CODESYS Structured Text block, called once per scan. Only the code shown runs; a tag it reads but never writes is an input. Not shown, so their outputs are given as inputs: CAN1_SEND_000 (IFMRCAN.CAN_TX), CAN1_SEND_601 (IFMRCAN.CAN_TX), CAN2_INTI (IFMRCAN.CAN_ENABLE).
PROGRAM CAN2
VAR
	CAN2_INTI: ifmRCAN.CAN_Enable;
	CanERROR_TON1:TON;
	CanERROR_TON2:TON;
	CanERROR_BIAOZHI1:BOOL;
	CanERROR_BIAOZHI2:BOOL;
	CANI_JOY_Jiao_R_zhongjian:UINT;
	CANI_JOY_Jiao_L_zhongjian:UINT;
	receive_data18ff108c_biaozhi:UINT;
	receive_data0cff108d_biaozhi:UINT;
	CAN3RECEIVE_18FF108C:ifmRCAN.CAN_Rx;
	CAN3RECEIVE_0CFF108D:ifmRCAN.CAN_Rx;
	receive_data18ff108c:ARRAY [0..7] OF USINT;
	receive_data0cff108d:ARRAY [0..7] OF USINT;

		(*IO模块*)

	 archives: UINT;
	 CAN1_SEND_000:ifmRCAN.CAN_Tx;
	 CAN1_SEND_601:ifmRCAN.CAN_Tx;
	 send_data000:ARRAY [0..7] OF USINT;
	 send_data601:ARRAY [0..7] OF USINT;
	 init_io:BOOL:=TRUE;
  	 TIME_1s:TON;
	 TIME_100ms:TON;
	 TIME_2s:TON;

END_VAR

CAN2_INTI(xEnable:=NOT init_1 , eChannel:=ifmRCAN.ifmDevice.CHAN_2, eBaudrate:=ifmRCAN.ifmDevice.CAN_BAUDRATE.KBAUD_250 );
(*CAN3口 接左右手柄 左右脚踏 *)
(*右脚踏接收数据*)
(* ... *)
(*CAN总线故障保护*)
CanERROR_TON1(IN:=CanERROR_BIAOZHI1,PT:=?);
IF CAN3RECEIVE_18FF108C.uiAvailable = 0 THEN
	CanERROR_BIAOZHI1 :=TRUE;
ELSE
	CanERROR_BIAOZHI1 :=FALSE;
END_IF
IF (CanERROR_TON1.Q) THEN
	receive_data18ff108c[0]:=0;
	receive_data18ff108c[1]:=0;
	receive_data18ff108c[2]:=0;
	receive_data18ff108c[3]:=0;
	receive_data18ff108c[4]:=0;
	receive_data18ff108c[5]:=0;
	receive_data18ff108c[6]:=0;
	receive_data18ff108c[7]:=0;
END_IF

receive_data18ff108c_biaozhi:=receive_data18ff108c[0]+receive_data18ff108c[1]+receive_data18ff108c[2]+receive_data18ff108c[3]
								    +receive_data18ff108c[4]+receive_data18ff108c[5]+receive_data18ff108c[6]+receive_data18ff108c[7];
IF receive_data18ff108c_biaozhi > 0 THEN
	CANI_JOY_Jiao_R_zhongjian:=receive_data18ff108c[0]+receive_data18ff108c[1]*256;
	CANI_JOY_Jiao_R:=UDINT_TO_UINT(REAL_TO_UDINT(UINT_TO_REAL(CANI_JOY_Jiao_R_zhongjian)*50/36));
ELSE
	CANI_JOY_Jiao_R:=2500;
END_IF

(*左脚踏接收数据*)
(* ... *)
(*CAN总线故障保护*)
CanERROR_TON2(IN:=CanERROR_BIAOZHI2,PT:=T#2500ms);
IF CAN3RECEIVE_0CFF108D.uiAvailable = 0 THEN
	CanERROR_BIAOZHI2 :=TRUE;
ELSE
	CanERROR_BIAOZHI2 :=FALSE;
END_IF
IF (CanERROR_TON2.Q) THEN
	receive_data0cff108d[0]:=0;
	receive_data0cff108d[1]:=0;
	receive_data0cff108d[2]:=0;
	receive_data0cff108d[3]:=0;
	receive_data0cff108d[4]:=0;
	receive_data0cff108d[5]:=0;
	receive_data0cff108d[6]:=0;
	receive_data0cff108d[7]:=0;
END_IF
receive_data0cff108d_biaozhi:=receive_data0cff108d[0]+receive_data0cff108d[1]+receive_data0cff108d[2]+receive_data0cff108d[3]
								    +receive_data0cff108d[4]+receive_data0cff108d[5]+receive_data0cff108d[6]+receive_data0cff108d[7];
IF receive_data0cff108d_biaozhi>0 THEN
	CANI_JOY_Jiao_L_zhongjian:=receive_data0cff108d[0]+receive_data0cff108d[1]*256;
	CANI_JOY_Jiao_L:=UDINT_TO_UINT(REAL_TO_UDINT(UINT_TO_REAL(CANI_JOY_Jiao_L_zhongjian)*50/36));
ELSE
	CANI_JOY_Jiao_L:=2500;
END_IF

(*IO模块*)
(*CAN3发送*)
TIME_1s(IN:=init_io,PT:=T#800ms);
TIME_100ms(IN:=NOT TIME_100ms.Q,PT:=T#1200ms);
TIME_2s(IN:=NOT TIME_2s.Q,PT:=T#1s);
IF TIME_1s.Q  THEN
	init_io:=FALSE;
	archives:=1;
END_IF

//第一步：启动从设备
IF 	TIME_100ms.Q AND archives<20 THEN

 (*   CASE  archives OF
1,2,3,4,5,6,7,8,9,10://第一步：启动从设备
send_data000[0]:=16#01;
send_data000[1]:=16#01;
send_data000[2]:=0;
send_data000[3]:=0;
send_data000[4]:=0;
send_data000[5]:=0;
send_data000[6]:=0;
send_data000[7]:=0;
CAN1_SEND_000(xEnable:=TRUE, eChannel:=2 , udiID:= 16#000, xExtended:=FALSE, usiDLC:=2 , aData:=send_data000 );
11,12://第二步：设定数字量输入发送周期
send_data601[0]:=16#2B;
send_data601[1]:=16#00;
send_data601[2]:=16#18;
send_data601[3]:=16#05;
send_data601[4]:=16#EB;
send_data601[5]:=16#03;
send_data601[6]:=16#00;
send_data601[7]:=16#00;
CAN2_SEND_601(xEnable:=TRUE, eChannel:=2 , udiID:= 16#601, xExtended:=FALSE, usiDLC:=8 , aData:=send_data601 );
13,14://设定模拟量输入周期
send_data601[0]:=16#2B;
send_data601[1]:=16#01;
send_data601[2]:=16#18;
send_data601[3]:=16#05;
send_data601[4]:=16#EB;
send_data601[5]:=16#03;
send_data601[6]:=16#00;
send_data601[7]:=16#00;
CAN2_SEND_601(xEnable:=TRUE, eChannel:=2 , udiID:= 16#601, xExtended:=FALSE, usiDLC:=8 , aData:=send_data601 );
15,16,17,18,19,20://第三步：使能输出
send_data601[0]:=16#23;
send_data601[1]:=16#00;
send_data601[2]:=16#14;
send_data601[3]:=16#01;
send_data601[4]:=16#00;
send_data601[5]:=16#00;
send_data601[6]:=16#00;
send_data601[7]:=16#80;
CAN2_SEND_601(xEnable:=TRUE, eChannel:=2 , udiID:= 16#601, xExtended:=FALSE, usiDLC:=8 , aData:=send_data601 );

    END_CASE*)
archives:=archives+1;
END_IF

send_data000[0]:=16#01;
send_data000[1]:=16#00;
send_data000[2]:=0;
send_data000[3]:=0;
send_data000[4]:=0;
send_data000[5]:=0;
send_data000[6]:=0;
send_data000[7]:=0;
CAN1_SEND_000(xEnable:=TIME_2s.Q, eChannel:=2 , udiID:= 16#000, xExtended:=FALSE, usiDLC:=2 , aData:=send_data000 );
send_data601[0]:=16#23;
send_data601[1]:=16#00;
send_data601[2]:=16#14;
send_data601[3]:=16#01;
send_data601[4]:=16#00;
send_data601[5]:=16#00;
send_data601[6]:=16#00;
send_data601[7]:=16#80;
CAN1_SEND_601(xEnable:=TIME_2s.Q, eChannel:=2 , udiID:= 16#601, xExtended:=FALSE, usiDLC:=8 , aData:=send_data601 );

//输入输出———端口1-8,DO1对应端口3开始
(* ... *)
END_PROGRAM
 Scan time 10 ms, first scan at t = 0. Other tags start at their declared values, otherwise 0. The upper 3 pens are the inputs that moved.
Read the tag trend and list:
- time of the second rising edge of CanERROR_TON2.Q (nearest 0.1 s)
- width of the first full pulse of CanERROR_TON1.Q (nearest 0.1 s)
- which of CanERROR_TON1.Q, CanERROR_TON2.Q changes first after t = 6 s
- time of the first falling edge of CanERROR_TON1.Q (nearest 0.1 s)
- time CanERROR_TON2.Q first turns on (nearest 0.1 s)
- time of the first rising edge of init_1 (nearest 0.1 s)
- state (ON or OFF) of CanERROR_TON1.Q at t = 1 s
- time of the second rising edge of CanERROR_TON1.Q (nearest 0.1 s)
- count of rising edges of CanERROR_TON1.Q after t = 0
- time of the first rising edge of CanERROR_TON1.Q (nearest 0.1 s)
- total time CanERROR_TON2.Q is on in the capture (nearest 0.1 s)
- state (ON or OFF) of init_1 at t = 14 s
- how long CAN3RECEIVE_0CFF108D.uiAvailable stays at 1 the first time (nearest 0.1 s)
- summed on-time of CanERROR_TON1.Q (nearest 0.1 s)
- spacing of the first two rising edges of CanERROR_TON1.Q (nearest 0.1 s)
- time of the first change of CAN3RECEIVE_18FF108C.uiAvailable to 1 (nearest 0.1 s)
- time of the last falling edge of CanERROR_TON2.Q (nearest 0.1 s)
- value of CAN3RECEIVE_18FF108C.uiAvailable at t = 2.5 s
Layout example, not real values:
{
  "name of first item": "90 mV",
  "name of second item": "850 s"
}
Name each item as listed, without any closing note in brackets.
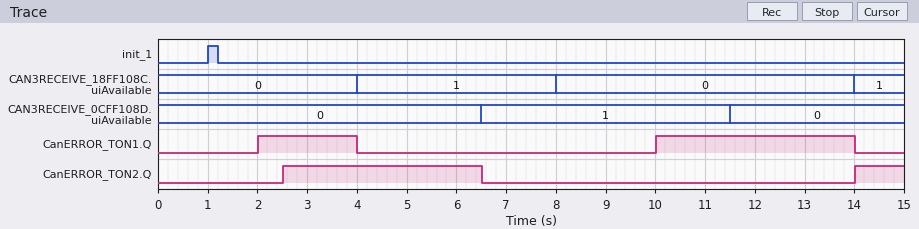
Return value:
{
  "time of the second rising edge of CanERROR_TON2.Q": "14.0 s",
  "width of the first full pulse of CanERROR_TON1.Q": "2.0 s",
  "which of CanERROR_TON1.Q, CanERROR_TON2.Q changes first after t = 6 s": "CanERROR_TON2.Q",
  "time of the first falling edge of CanERROR_TON1.Q": "4.0 s",
  "time CanERROR_TON2.Q first turns on": "2.5 s",
  "time of the first rising edge of init_1": "1.0 s",
  "state (ON or OFF) of CanERROR_TON1.Q at t = 1 s": "OFF",
  "time of the second rising edge of CanERROR_TON1.Q": "10.0 s",
  "count of rising edges of CanERROR_TON1.Q after t = 0": "2",
  "time of the first rising edge of CanERROR_TON1.Q": "2.0 s",
  "total time CanERROR_TON2.Q is on in the capture": "5.0 s",
  "state (ON or OFF) of init_1 at t = 14 s": "OFF",
  "how long CAN3RECEIVE_0CFF108D.uiAvailable stays at 1 the first time": "5.0 s",
  "summed on-time of CanERROR_TON1.Q": "6.0 s",
  "spacing of the first two rising edges of CanERROR_TON1.Q": "8.0 s",
  "time of the first change of CAN3RECEIVE_18FF108C.uiAvailable to 1": "4.0 s",
  "time of the last falling edge of CanERROR_TON2.Q": "6.5 s",
  "value of CAN3RECEIVE_18FF108C.uiAvailable at t = 2.5 s": "0"
}
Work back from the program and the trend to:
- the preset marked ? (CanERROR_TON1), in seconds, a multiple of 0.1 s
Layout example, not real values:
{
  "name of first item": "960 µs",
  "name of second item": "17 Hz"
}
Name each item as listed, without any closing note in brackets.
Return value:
{
  "the preset marked ? (CanERROR_TON1), in seconds, a multiple of 0.1 s": "2.0 s"
}
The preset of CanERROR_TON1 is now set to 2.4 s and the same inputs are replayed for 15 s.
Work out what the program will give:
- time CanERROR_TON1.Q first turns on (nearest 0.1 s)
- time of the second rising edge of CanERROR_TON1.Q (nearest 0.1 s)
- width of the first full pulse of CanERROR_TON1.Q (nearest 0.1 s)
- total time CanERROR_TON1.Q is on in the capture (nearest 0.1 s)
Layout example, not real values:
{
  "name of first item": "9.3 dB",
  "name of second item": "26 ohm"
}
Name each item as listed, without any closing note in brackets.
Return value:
{
  "time CanERROR_TON1.Q first turns on": "2.4 s",
  "time of the second rising edge of CanERROR_TON1.Q": "10.4 s",
  "width of the first full pulse of CanERROR_TON1.Q": "1.6 s",
  "total time CanERROR_TON1.Q is on in the capture": "5.2 s"
}
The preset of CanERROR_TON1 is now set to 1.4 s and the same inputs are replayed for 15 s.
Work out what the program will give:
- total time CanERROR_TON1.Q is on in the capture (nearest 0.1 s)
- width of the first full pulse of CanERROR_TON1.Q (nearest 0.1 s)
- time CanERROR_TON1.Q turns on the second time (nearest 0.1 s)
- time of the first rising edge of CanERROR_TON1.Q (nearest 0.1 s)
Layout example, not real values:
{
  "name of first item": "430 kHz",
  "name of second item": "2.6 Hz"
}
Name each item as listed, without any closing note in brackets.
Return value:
{
  "total time CanERROR_TON1.Q is on in the capture": "7.2 s",
  "width of the first full pulse of CanERROR_TON1.Q": "2.6 s",
  "time CanERROR_TON1.Q turns on the second time": "9.4 s",
  "time of the first rising edge of CanERROR_TON1.Q": "1.4 s"
}
